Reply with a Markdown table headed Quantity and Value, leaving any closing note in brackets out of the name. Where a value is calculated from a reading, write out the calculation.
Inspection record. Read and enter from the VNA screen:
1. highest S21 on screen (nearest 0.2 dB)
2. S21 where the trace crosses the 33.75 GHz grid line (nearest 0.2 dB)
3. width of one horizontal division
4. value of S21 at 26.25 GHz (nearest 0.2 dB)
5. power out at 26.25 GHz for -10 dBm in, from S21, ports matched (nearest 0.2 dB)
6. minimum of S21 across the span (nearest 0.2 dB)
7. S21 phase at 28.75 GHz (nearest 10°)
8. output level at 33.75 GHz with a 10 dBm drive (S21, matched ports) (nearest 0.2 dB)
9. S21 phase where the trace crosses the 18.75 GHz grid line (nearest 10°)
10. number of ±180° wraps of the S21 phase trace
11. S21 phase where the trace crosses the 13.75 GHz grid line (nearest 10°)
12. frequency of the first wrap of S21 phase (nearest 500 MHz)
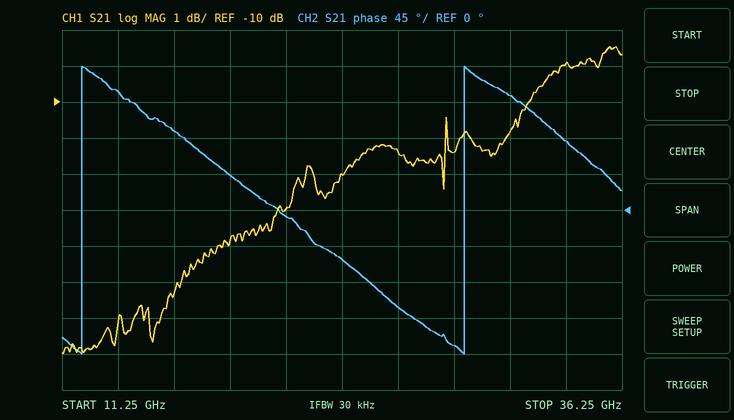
| Quantity | Value |
|---|---|
| highest S21 on screen | -8.4 dB |
| S21 where the trace crosses the 33.75 GHz grid line | -9.0 dB |
| width of one horizontal division | 2.5 GHz |
| value of S21 at 26.25 GHz | -11.4 dB |
| power out at 26.25 GHz for -10 dBm in, from S21, ports matched | -10 dBm + (-11.4 dB) = -21.4 dBm |
| minimum of S21 across the span | -17.0 dB |
| S21 phase at 28.75 GHz | -170° |
| output level at 33.75 GHz with a 10 dBm drive (S21, matched ports) | 10 dBm + (-9.0 dB) = 1.0 dBm |
| S21 phase where the trace crosses the 18.75 GHz grid line | 40° |
| number of ±180° wraps of the S21 phase trace | 2 |
| S21 phase where the trace crosses the 13.75 GHz grid line | 150° |
| frequency of the first wrap of S21 phase | 12.0 GHz |
